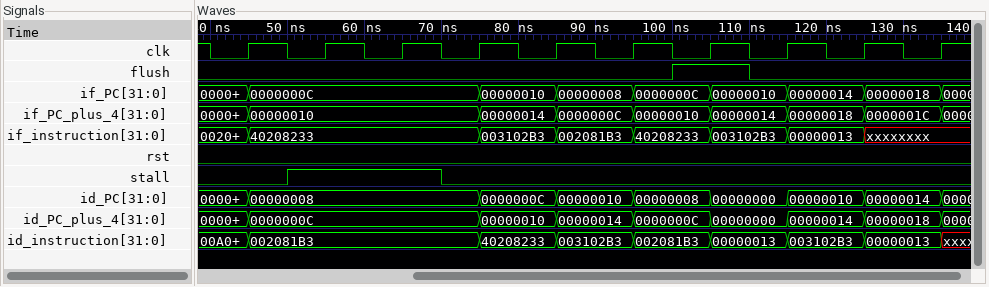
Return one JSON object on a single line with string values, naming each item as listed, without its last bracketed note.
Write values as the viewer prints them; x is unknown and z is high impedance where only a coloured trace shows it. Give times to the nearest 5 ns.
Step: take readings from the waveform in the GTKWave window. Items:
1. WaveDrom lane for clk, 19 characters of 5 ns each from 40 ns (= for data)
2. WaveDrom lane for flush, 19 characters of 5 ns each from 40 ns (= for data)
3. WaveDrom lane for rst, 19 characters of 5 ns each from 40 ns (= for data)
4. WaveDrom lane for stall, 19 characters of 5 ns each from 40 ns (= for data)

{"WaveDrom lane for clk, 19 characters of 5 ns each from 40 ns": "{name: 'clk', wave: '0101010101010101010'}", "WaveDrom lane for flush, 19 characters of 5 ns each from 40 ns": "{name: 'flush', wave: '0...........1.0....'}", "WaveDrom lane for rst, 19 characters of 5 ns each from 40 ns": "{name: 'rst', wave: '0..................'}", "WaveDrom lane for stall, 19 characters of 5 ns each from 40 ns": "{name: 'stall', wave: '0.1...0............'}"}
